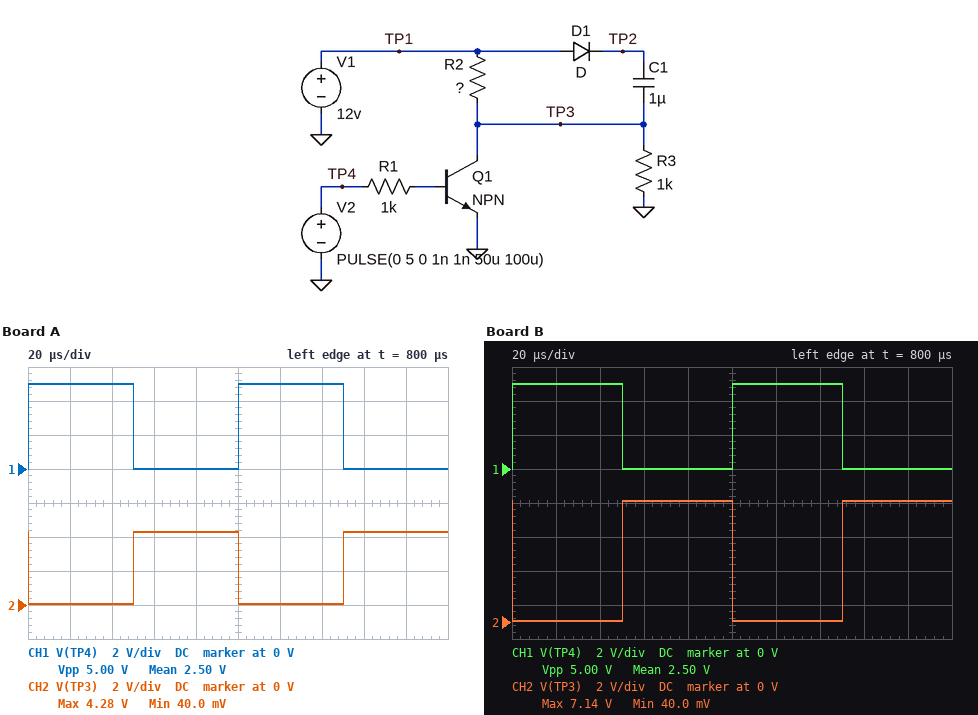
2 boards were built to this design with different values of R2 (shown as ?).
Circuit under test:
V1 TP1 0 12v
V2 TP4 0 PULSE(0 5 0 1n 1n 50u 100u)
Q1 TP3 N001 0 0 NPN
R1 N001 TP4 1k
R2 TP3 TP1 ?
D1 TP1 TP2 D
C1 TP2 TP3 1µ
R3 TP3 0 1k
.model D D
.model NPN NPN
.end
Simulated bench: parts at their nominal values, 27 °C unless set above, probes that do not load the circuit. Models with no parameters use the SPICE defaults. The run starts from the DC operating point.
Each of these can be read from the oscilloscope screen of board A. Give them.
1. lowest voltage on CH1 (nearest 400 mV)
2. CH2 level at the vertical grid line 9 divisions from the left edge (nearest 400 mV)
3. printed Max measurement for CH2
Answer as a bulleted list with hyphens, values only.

- 0 V
- 4.4 V
- 4.28 V
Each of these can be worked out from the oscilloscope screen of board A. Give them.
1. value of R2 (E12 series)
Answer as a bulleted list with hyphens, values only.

- 1.8 kΩ
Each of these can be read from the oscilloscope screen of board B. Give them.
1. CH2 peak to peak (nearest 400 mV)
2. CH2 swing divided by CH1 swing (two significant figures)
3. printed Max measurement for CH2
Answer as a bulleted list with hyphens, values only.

- 7.2 V
- 1.4
- 7.14 V
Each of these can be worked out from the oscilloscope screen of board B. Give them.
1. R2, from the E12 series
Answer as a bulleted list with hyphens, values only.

- 680 Ω
